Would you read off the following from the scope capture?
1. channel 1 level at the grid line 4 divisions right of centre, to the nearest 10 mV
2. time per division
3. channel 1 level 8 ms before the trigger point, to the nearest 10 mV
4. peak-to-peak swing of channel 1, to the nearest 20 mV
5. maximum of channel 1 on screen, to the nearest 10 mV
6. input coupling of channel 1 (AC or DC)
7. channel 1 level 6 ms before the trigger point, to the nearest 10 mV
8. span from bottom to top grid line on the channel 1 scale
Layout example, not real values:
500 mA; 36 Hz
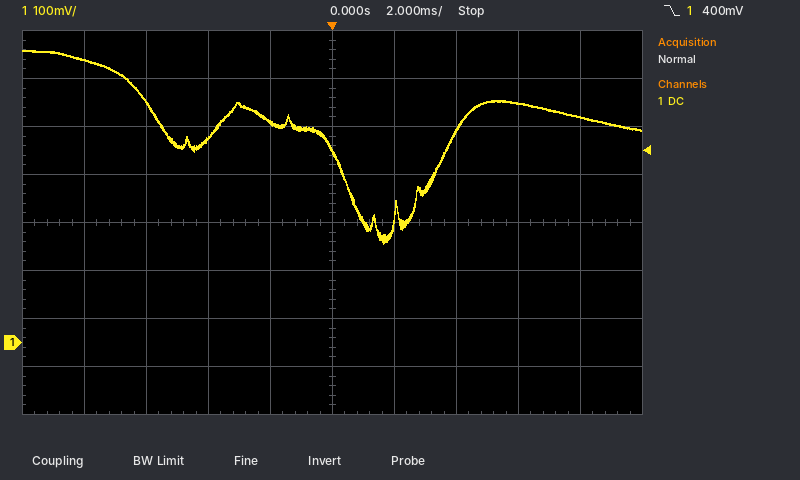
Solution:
470 mV; 2 ms; 590 mV; 400 mV; 610 mV; DC; 500 mV; 800 mV
